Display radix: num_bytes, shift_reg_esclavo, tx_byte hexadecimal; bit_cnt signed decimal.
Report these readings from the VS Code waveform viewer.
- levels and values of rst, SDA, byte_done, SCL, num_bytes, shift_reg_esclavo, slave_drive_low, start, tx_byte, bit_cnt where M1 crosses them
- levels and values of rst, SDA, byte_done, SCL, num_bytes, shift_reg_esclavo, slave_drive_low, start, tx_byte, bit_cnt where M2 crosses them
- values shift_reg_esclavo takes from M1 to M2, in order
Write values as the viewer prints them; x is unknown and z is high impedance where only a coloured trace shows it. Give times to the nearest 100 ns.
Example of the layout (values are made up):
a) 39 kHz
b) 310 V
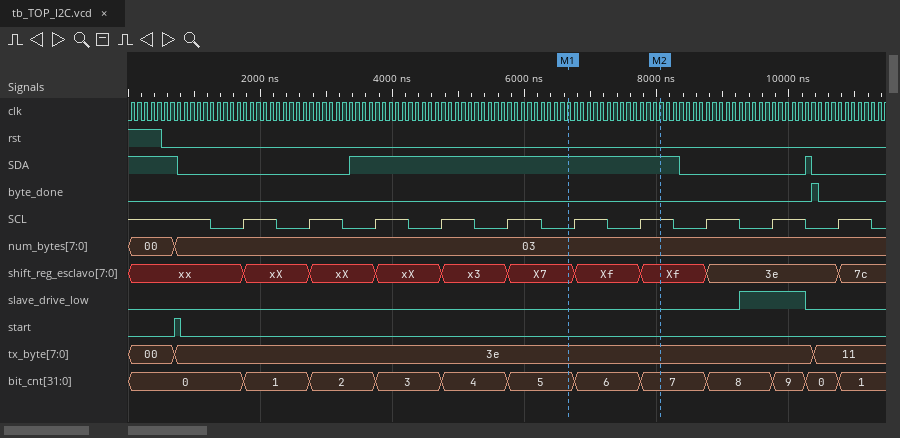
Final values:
a) rst=0, SDA=1, byte_done=0, SCL=0, num_bytes=03, shift_reg_esclavo=X7, slave_drive_low=0, start=0, tx_byte=3e, bit_cnt=5
b) rst=0, SDA=1, byte_done=0, SCL=z, num_bytes=03, shift_reg_esclavo=Xf, slave_drive_low=0, start=0, tx_byte=3e, bit_cnt=7
c) X7, Xf, Xf
